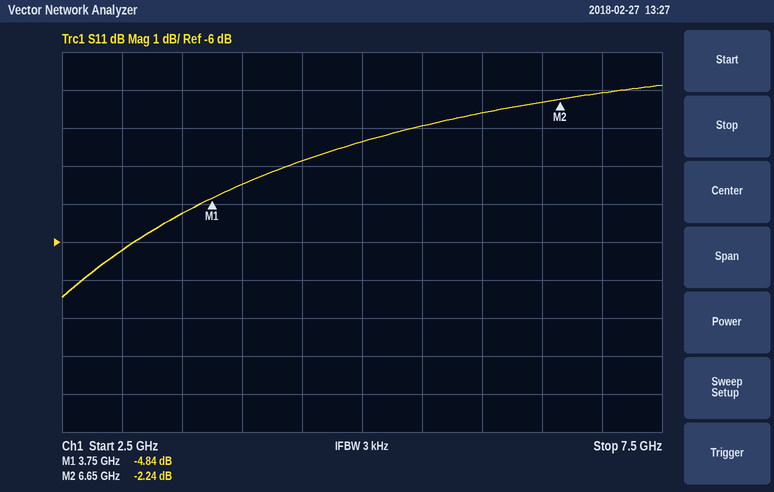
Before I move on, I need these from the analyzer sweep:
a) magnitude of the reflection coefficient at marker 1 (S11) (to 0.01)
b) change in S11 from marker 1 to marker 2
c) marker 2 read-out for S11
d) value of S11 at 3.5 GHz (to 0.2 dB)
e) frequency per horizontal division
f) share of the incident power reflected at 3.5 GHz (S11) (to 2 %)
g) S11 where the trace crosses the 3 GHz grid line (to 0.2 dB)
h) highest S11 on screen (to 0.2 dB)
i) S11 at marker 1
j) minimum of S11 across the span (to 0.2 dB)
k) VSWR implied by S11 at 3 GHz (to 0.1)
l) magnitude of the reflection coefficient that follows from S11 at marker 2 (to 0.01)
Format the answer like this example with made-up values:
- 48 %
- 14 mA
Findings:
- 0.57
- 2.60 dB
- -2.24 dB
- -5.2 dB
- 500 MHz
- 30 %
- -6.2 dB
- -1.8 dB
- -4.84 dB
- -7.4 dB
- 2.9
- 0.77
